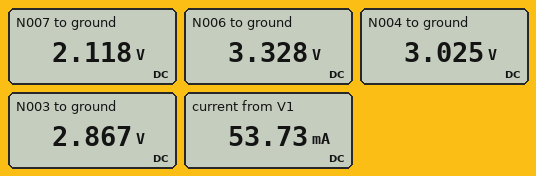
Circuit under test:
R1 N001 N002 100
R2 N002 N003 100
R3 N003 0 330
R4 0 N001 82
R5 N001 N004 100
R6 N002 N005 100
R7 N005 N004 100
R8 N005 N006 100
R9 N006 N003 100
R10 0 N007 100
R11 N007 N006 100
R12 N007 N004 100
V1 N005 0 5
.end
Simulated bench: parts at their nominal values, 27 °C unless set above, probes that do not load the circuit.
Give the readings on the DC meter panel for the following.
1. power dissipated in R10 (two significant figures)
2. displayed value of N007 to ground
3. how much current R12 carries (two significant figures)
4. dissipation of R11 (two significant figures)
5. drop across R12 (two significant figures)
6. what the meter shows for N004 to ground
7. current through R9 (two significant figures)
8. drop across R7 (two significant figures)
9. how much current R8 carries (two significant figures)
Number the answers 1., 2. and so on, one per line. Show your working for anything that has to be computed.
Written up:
1. (2.118 V)^2 / 100 Ω = 45 mW
2. 2.118 V
3. (3.025 V - 2.118 V) / 100 Ω = 9.1 mA
4. (3.328 V - 2.118 V)^2 / 100 Ω = 15 mW
5. 3.025 V - 2.118 V = 910 mV
6. 3.025 V
7. (3.328 V - 2.867 V) / 100 Ω = 4.6 mA
8. 5 V - 3.025 V = 2.0 V
9. (5 V - 3.328 V) / 100 Ω = 17 mA
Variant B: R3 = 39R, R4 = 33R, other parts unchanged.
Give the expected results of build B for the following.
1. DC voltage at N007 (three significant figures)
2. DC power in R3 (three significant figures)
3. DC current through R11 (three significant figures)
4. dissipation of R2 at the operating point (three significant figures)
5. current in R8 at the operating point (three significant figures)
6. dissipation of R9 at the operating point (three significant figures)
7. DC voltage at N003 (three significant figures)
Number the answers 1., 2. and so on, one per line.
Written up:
1. 1.72 V
2. 30.3 mW
3. 8.80 mA
4. 16.1 mW
5. 24.0 mA
6. 23.0 mW
7. 1.09 V
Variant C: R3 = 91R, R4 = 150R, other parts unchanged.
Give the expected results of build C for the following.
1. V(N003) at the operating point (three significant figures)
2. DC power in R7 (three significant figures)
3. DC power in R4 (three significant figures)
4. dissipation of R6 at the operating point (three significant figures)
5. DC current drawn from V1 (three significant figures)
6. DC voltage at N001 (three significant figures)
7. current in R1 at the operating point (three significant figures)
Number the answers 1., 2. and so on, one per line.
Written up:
1. 1.97 V
2. 35.1 mW
3. 36.4 mW
4. 36.0 mW
5. 57.7 mA
6. 2.34 V
7. 7.66 mA
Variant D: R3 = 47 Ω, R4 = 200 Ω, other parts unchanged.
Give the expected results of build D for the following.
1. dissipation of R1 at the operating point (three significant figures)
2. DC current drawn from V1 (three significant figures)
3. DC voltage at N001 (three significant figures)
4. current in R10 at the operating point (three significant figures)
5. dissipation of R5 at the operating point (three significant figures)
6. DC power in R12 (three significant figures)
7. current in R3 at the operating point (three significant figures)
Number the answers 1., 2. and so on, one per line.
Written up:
1. 2.60 mW
2. 61.4 mA
3. 2.43 V
4. 19.7 mA
5. 4.97 mW
6. 13.5 mW
7. 29.5 mA
